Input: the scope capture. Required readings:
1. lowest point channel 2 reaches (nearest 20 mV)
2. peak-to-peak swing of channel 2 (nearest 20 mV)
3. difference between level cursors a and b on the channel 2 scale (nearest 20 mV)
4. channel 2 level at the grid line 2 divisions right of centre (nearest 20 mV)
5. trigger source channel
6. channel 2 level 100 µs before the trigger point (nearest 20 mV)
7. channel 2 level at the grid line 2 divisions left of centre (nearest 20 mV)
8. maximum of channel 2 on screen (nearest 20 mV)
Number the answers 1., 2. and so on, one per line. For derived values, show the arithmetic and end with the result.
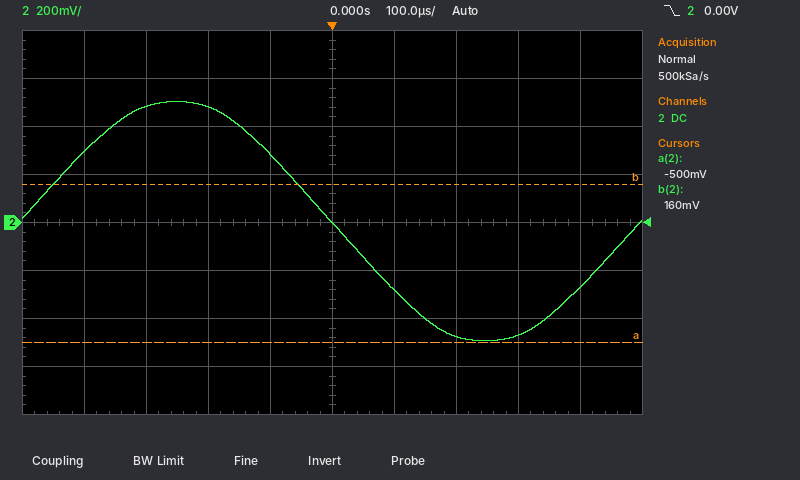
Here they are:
1. -500 mV
2. 500 mV − (-500 mV) = 1.00 V
3. 660 mV
4. -480 mV
5. channel 2
6. 280 mV
7. 480 mV
8. 500 mV
